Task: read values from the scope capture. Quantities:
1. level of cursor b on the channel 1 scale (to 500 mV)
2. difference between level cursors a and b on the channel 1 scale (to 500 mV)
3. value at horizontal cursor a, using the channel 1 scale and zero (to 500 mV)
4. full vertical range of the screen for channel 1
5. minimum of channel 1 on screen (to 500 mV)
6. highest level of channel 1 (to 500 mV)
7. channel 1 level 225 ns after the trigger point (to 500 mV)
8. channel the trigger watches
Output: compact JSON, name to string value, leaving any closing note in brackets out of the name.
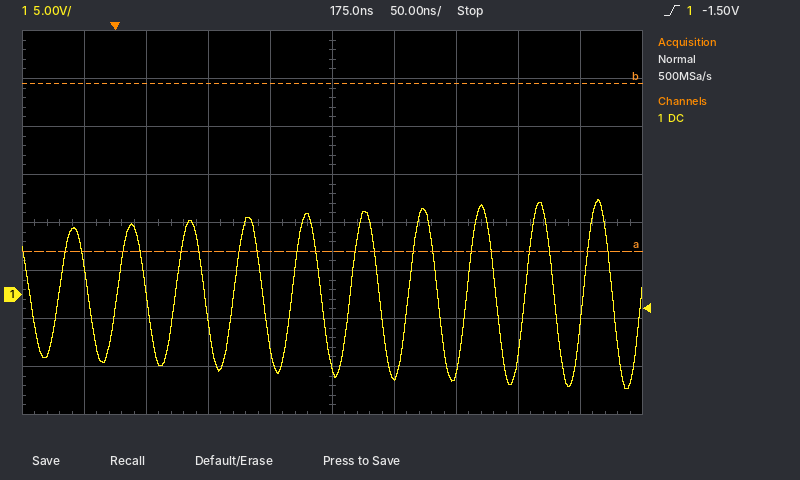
{"level of cursor b on the channel 1 scale": "22.0 V", "difference between level cursors a and b on the channel 1 scale": "17.5 V", "value at horizontal cursor a, using the channel 1 scale and zero": "4.5 V", "full vertical range of the screen for channel 1": "40 V", "minimum of channel 1 on screen": "-10.0 V", "highest level of channel 1": "10.0 V", "channel 1 level 225 ns after the trigger point": "-8.5 V", "channel the trigger watches": "channel 1"}
